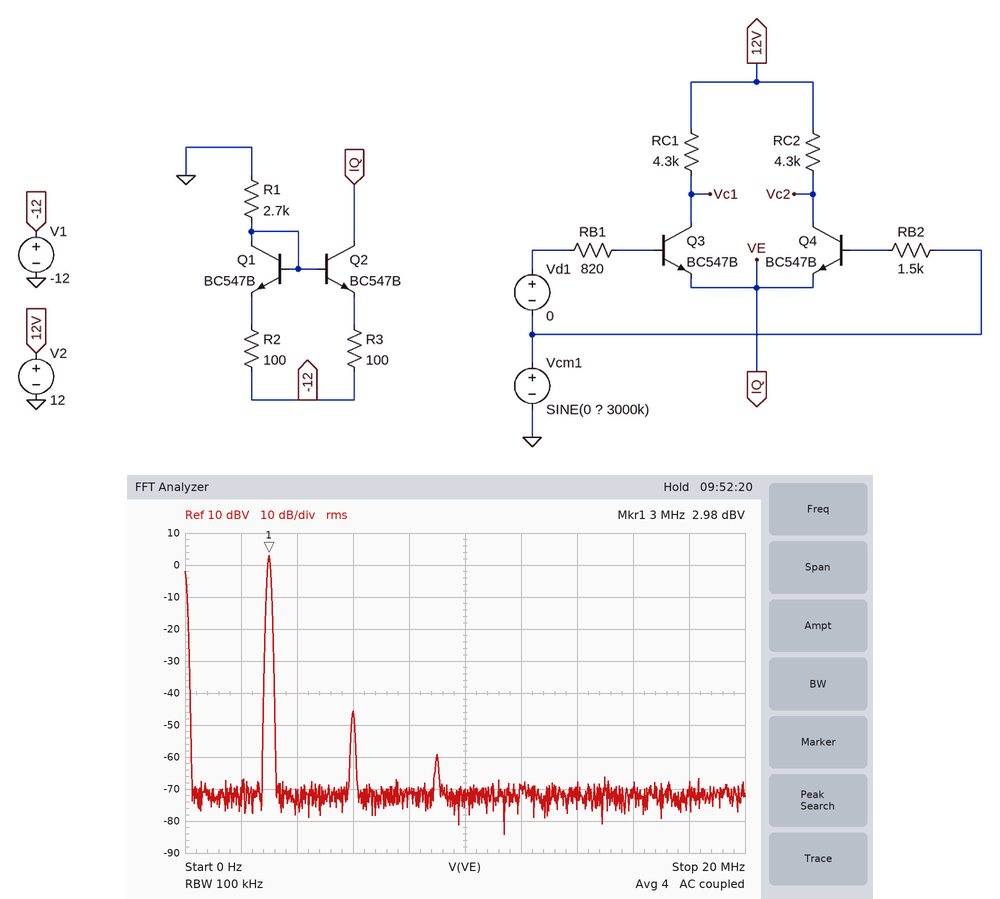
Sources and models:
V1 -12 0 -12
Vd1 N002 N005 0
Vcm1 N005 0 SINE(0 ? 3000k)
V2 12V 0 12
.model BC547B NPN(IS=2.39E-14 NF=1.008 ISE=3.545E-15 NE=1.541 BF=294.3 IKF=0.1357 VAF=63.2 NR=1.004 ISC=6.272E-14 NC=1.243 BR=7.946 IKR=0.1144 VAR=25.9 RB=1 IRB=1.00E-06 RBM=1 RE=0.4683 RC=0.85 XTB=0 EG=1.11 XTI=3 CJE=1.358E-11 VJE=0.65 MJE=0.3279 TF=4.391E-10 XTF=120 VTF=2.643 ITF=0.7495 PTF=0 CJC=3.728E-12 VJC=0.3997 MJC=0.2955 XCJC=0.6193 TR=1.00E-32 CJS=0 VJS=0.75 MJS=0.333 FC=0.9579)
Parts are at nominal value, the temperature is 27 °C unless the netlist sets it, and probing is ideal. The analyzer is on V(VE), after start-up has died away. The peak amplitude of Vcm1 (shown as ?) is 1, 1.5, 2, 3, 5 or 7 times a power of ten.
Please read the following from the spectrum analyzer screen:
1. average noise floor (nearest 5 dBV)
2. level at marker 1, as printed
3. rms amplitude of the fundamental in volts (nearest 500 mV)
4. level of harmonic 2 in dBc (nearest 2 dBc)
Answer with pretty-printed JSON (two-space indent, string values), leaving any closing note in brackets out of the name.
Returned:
{
  "average noise floor": "-70 dBV",
  "level at marker 1, as printed": "2.98 dBV",
  "rms amplitude of the fundamental in volts": "1.5 V",
  "level of harmonic 2 in dBc": "-48 dBc"
}
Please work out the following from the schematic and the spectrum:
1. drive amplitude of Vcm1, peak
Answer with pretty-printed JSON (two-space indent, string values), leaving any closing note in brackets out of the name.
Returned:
{
  "drive amplitude of Vcm1, peak": "2 V"
}
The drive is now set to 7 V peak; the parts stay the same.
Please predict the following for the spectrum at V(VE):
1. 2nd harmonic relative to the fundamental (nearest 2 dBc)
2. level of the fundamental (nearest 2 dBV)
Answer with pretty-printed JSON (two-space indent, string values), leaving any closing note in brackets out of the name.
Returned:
{
  "2nd harmonic relative to the fundamental": "-30 dBc",
  "level of the fundamental": "14 dBV"
}
